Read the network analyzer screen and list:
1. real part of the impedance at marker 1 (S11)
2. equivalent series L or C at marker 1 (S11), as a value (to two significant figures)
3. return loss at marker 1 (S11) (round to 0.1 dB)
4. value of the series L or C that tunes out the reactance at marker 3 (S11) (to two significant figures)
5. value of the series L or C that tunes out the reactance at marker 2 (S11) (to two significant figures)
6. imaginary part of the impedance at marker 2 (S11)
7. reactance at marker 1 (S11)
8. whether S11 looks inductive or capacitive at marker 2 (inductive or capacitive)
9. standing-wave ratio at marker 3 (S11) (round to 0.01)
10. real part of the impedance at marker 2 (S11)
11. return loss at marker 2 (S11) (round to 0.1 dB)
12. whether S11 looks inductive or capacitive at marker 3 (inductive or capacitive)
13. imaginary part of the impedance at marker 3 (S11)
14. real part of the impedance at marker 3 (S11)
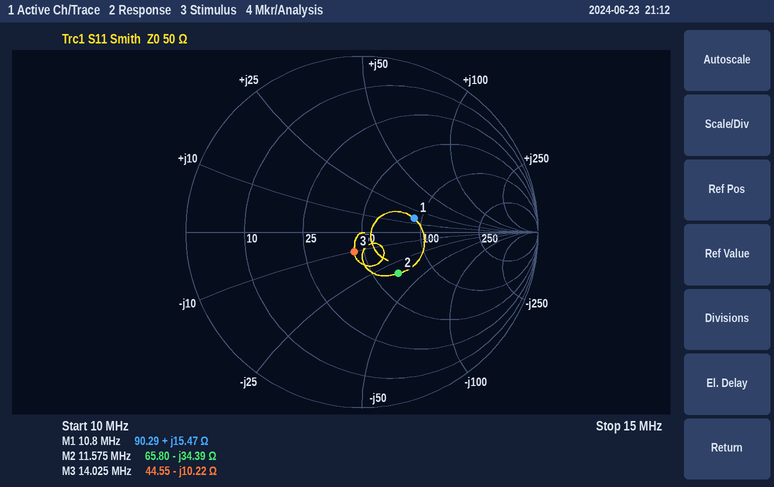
90.29 Ω
230 nH
10.3 dB
120 nH
470 nH
-34.39 Ω
+15.47 Ω
capacitive
1.28
65.80 Ω
10.1 dB
capacitive
-10.22 Ω
44.55 Ω
